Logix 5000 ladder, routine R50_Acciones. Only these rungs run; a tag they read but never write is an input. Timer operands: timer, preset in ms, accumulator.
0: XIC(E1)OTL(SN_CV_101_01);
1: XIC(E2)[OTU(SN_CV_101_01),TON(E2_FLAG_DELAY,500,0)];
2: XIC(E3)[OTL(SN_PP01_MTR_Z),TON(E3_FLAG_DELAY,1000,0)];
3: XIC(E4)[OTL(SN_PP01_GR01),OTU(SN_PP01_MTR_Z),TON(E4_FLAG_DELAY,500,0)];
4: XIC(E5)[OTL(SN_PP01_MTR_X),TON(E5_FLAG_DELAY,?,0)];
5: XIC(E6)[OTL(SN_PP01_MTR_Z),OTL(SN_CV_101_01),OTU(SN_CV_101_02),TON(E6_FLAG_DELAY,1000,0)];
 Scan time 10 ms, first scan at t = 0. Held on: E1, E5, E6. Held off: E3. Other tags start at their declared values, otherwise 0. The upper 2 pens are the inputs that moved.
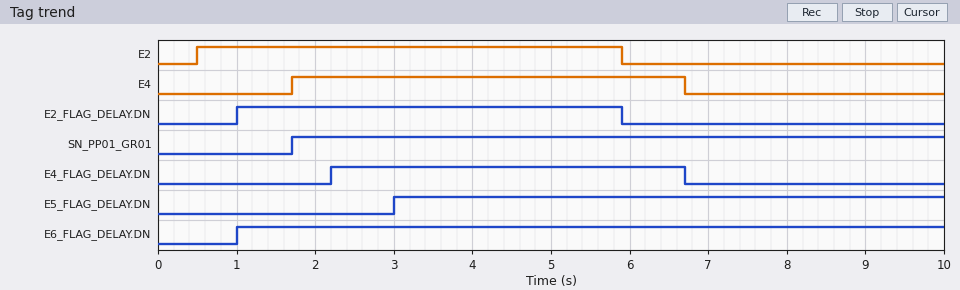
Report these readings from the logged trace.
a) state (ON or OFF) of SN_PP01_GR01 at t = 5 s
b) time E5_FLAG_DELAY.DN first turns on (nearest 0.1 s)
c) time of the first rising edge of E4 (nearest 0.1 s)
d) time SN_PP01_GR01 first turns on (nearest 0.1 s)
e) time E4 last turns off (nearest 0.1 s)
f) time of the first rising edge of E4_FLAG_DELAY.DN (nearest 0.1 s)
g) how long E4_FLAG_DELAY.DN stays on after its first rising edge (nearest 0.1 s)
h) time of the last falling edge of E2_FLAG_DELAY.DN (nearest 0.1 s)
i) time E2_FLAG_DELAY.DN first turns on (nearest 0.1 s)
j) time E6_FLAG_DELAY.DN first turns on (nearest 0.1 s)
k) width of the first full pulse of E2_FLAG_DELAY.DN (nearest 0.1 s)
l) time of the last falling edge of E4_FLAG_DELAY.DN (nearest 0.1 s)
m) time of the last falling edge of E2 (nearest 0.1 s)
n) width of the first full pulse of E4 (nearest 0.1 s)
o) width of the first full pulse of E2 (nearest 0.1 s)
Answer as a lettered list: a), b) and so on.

a) ON
b) 3.0 s
c) 1.7 s
d) 1.7 s
e) 6.7 s
f) 2.2 s
g) 4.5 s
h) 5.9 s
i) 1.0 s
j) 1.0 s
k) 4.9 s
l) 6.7 s
m) 5.9 s
n) 5.0 s
o) 5.4 s
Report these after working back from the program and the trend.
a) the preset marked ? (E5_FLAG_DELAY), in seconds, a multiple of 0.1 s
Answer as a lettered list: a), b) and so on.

a) 3.0 s
